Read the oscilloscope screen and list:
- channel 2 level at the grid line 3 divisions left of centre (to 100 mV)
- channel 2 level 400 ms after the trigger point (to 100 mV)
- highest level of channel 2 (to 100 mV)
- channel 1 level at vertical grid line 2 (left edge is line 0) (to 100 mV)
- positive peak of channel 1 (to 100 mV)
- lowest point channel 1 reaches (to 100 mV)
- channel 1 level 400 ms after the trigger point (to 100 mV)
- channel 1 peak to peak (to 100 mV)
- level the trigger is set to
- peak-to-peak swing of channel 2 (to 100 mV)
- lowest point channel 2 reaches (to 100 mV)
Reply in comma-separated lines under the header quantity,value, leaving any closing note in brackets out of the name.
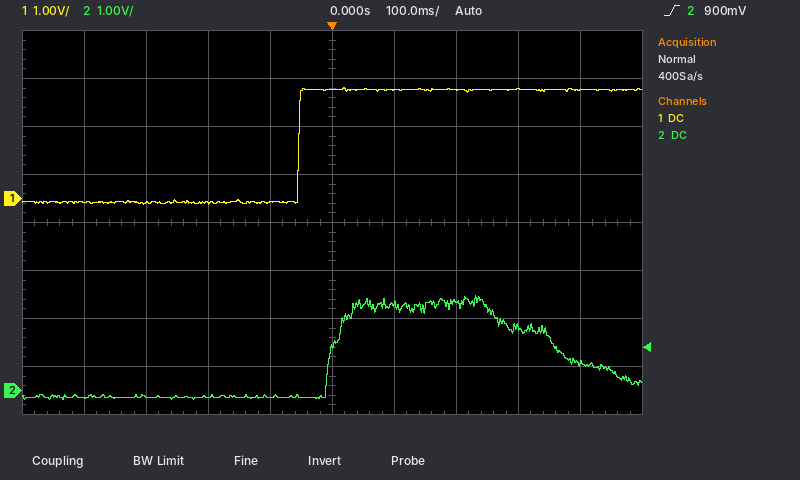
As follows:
quantity,value
channel 2 level at the grid line 3 divisions left of centre,-100 mV
channel 2 level 400 ms after the trigger point,600 mV
highest level of channel 2,2.0 V
channel 1 level at vertical grid line 2 (left edge is line 0),-100 mV
positive peak of channel 1,2.3 V
lowest point channel 1 reaches,-100 mV
channel 1 level 400 ms after the trigger point,2.3 V
channel 1 peak to peak,2.4 V
level the trigger is set to,900 mV
peak-to-peak swing of channel 2,2.2 V
lowest point channel 2 reaches,-200 mV
